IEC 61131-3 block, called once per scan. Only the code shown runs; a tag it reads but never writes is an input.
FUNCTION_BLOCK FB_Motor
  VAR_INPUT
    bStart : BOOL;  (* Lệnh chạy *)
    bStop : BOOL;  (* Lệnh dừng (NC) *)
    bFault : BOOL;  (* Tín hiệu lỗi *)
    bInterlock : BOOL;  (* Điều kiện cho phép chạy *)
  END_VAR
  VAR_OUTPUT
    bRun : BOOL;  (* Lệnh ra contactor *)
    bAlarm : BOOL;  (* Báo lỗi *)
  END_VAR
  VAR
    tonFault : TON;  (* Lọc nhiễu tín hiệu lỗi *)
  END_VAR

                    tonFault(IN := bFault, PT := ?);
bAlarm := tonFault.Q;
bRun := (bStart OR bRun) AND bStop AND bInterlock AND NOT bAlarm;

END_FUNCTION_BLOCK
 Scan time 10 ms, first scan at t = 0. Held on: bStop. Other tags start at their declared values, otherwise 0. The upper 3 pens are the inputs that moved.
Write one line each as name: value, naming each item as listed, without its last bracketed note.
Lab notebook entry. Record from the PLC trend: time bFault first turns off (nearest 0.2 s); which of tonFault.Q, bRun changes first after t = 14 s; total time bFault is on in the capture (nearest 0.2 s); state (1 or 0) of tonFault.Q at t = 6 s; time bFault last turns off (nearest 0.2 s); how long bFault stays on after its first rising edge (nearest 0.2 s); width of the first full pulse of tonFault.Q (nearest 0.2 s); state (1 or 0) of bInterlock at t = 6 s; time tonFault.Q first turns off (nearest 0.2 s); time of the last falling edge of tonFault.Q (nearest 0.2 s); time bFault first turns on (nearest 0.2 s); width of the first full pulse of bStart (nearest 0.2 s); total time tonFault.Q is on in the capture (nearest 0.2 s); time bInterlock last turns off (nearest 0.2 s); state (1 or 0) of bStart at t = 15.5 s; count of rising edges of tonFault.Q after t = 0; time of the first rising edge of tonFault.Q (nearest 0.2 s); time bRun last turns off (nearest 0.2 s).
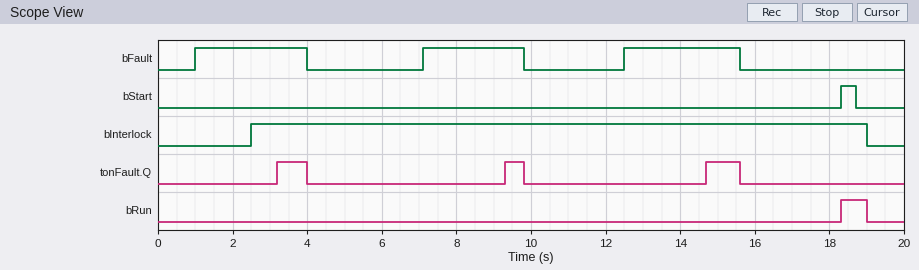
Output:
time bFault first turns off: 4.0 s
which of tonFault.Q, bRun changes first after t = 14 s: tonFault.Q
total time bFault is on in the capture: 8.8 s
state (1 or 0) of tonFault.Q at t = 6 s: 0
time bFault last turns off: 15.6 s
how long bFault stays on after its first rising edge: 3.0 s
width of the first full pulse of tonFault.Q: 0.8 s
state (1 or 0) of bInterlock at t = 6 s: 1
time tonFault.Q first turns off: 4.0 s
time of the last falling edge of tonFault.Q: 15.6 s
time bFault first turns on: 1.0 s
width of the first full pulse of bStart: 0.4 s
total time tonFault.Q is on in the capture: 2.2 s
time bInterlock last turns off: 19.0 s
state (1 or 0) of bStart at t = 15.5 s: 0
count of rising edges of tonFault.Q after t = 0: 3
time of the first rising edge of tonFault.Q: 3.2 s
time bRun last turns off: 19.0 s
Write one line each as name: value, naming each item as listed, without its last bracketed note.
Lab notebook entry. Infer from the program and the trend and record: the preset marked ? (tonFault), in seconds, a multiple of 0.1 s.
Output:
the preset marked ? (tonFault), in seconds, a multiple of 0.1 s: 2.2 s
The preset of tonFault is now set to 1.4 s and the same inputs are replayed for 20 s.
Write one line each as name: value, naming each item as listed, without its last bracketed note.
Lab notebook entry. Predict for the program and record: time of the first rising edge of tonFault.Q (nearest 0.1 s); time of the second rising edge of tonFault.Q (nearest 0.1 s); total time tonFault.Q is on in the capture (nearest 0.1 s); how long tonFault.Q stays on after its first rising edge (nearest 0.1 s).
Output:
time of the first rising edge of tonFault.Q: 2.4 s
time of the second rising edge of tonFault.Q: 8.5 s
total time tonFault.Q is on in the capture: 4.6 s
how long tonFault.Q stays on after its first rising edge: 1.6 s
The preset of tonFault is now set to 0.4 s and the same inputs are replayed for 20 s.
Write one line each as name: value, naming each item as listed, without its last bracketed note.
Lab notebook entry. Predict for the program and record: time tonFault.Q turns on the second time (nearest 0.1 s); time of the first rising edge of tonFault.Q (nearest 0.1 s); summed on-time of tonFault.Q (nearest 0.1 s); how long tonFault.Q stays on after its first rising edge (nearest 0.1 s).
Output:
time tonFault.Q turns on the second time: 7.5 s
time of the first rising edge of tonFault.Q: 1.4 s
summed on-time of tonFault.Q: 7.6 s
how long tonFault.Q stays on after its first rising edge: 2.6 s
